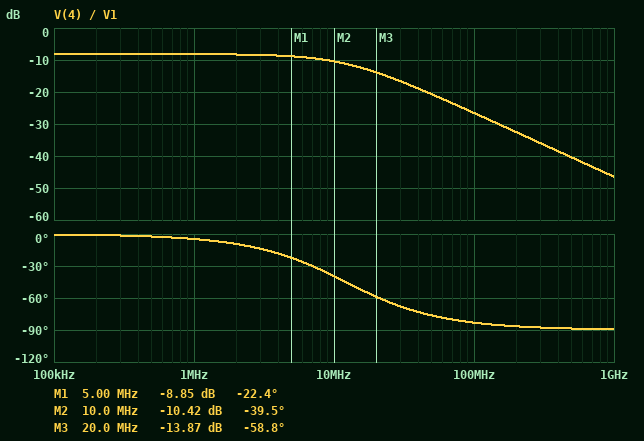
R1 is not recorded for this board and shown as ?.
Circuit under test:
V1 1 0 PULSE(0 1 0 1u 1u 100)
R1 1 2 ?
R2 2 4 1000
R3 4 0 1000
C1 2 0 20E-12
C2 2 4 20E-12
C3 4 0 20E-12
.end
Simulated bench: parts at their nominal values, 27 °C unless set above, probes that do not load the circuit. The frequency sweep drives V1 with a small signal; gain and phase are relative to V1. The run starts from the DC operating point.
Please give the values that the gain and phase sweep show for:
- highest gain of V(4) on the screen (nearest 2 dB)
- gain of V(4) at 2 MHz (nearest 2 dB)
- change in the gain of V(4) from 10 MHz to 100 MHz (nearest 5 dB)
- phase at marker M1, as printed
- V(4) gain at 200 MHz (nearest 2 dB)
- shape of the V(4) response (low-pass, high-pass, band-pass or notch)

-8 dB
-8 dB
-15 dB
-22.4 deg
-32 dB
low-pass
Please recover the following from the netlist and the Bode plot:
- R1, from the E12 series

560 Ω
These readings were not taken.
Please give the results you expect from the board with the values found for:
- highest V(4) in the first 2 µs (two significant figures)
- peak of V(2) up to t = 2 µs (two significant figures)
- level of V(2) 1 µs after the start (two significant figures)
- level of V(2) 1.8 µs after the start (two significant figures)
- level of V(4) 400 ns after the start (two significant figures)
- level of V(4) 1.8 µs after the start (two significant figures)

390 mV
780 mV
770 mV
780 mV
150 mV
390 mV
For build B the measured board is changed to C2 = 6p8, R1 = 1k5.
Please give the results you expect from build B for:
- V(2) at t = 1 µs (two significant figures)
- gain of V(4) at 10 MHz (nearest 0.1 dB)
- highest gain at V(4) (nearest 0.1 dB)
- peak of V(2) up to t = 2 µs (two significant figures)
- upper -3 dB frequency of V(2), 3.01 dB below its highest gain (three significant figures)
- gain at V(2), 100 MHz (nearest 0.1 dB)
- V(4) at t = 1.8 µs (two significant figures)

560 mV
-17.3 dB
-10.9 dB
570 mV
6.87 MHz
-27.5 dB
290 mV
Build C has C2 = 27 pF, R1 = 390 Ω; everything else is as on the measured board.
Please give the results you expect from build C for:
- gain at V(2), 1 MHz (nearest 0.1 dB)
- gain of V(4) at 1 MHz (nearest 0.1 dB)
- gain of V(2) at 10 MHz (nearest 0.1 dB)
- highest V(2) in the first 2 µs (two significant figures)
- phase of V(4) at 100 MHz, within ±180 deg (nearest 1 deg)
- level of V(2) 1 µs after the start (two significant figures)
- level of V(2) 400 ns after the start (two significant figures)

-1.6 dB
-7.6 dB
-3.1 dB
840 mV
-81 deg
830 mV
330 mV
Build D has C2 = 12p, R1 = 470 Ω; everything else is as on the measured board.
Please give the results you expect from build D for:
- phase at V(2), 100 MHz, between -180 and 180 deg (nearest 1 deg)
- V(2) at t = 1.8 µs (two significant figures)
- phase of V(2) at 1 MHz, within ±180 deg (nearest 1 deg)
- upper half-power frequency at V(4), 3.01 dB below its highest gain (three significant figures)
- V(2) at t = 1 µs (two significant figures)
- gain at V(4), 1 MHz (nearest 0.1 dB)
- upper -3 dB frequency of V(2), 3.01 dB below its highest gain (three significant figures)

-81 deg
810 mV
-4 deg
10.8 MHz
800 mV
-7.9 dB
15.0 MHz
